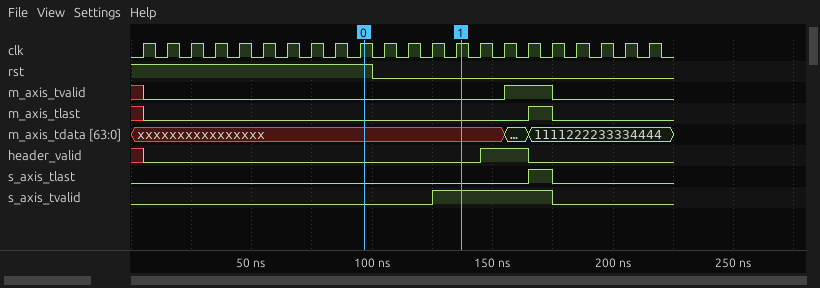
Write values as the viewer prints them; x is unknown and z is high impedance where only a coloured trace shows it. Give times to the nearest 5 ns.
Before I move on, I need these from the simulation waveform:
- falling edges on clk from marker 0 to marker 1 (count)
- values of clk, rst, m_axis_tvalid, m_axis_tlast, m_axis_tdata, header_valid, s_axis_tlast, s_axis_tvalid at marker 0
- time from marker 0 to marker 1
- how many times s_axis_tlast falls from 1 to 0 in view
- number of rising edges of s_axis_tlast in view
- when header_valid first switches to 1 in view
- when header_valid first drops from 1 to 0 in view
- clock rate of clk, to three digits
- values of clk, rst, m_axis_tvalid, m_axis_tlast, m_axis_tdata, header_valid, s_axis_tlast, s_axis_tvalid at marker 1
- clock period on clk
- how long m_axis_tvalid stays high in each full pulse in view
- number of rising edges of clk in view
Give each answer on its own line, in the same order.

4
clk=1, rst=1, m_axis_tvalid=0, m_axis_tlast=0, m_axis_tdata=xxxxxxxxxxxxxxxx, header_valid=0, s_axis_tlast=0, s_axis_tvalid=0
40 ns
1
1
145 ns
165 ns
100 MHz
clk=1, rst=0, m_axis_tvalid=0, m_axis_tlast=0, m_axis_tdata=xxxxxxxxxxxxxxxx, header_valid=0, s_axis_tlast=0, s_axis_tvalid=1
10 ns
20 ns
22
